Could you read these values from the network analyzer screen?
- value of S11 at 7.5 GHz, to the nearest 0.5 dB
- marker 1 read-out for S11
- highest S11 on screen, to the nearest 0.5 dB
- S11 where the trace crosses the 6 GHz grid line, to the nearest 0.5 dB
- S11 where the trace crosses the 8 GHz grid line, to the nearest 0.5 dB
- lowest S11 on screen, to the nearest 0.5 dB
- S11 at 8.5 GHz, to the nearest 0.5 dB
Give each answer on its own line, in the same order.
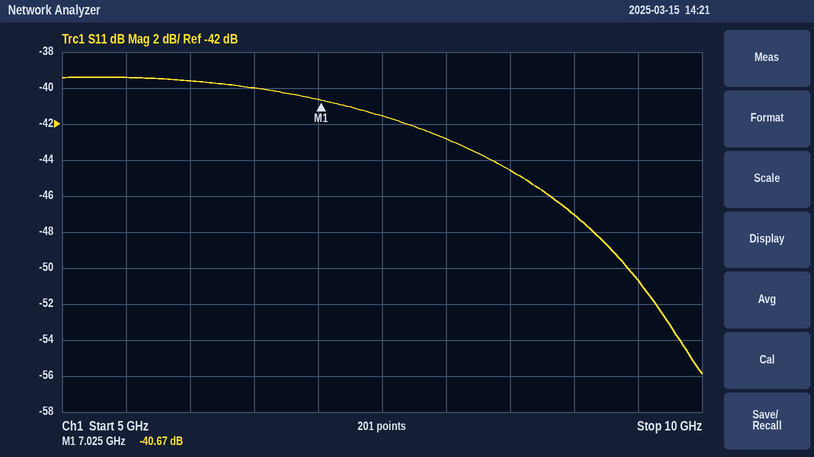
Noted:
-41.5 dB
-40.67 dB
-39.5 dB
-39.5 dB
-43.0 dB
-56.0 dB
-44.5 dB
